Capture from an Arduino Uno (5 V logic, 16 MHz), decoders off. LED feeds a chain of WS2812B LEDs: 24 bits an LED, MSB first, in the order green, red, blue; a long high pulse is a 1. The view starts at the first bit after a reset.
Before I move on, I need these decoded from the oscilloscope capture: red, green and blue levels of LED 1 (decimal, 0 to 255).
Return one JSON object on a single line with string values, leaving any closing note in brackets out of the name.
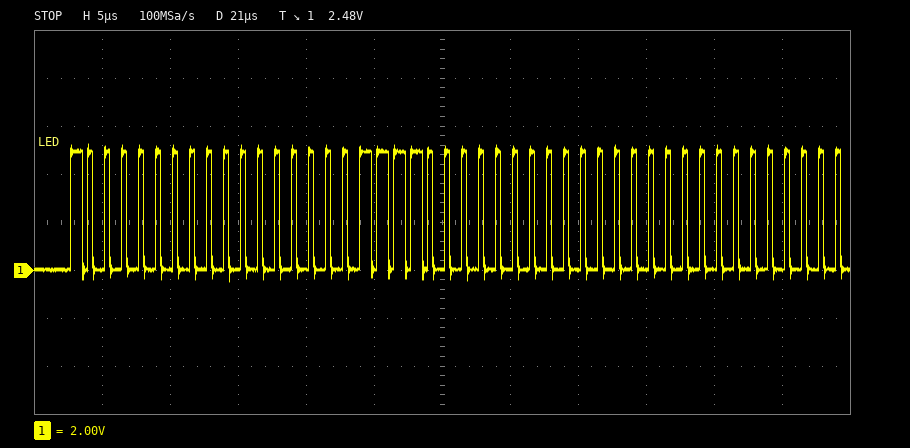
{"red, green and blue levels of LED 1": "0, 128, 120"}
